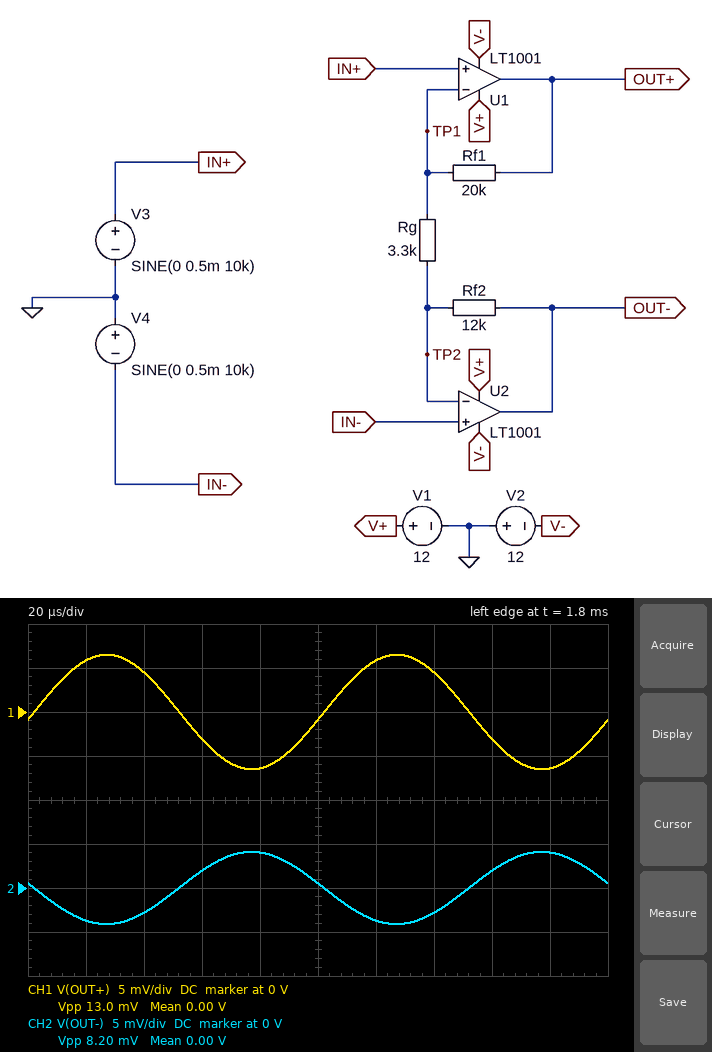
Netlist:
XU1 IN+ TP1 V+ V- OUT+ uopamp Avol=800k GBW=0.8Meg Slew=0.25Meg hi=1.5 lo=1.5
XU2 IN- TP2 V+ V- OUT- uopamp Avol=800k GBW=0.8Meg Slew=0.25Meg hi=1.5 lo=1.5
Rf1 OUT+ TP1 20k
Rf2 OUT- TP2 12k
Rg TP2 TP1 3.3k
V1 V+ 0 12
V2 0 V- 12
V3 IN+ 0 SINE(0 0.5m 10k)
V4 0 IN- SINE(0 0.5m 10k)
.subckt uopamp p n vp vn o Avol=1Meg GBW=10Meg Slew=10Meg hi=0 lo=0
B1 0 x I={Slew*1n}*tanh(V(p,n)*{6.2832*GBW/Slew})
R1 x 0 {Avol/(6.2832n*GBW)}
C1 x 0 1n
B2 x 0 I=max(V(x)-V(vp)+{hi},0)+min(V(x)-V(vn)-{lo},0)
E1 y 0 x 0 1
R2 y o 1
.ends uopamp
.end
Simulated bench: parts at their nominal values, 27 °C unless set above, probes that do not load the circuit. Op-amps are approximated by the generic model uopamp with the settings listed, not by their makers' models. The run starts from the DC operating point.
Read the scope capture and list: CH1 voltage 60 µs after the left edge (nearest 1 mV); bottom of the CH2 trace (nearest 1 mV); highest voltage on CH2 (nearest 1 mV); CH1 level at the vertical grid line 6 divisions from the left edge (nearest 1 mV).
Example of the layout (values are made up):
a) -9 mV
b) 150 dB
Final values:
a) -3 mV
b) -4 mV
c) 4 mV
d) 6 mV
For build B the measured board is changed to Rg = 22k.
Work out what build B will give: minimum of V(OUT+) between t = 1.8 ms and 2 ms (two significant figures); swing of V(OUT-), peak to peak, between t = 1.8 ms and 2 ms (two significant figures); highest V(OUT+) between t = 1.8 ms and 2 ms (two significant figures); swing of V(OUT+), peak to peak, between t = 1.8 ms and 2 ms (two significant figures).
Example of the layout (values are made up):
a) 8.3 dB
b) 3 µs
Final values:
a) -1.4 mV
b) 2.1 mV
c) 1.4 mV
d) 2.8 mV
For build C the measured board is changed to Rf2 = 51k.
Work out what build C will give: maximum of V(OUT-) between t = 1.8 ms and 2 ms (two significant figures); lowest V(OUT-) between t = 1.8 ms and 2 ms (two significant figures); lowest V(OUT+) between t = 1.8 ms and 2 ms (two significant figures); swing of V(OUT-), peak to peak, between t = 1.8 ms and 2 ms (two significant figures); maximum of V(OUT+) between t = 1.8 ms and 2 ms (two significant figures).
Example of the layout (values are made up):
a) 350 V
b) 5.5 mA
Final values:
a) 15 mV
b) -15 mV
c) -6.3 mV
d) 31 mV
e) 6.3 mV
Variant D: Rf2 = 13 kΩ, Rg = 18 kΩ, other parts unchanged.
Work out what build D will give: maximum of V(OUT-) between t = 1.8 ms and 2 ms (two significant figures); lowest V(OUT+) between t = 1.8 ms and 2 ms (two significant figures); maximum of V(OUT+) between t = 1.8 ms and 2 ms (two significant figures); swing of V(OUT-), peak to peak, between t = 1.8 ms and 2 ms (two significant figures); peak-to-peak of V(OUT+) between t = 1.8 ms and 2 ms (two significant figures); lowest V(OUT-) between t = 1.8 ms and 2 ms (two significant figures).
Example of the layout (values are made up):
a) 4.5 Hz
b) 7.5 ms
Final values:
a) 1.2 mV
b) -1.6 mV
c) 1.6 mV
d) 2.4 mV
e) 3.2 mV
f) -1.2 mV
